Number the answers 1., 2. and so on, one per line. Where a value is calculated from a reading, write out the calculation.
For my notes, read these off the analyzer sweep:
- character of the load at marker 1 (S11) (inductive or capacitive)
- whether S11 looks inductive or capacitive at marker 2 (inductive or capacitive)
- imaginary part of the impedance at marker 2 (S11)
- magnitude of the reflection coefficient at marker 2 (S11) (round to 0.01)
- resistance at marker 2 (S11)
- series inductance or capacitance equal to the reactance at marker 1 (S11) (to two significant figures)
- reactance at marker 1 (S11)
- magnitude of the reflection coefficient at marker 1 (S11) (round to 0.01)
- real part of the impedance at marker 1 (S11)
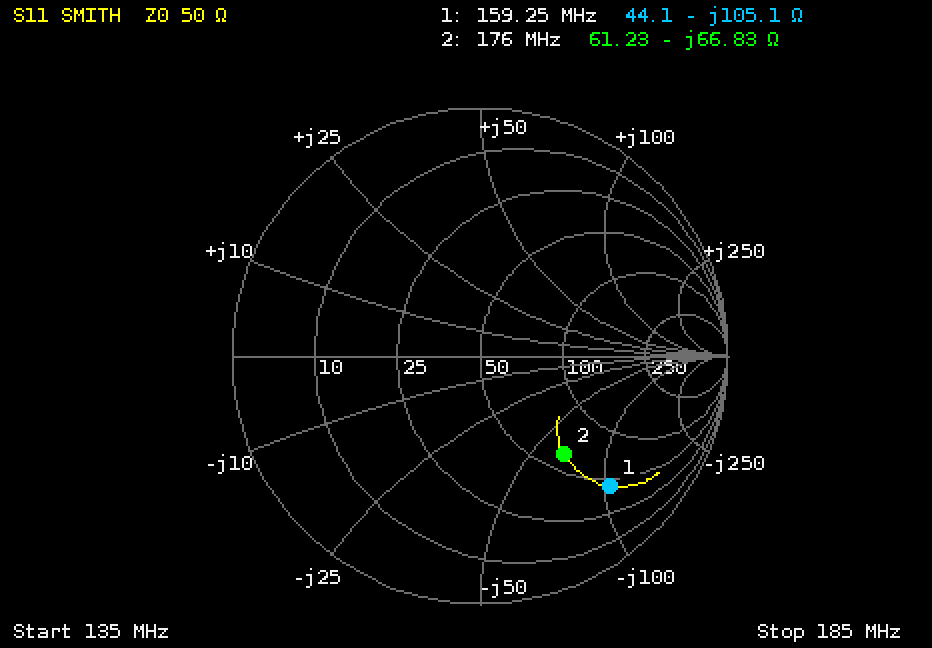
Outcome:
1. capacitive
2. capacitive
3. -66.83 Ω
4. 0.52
5. 61.23 Ω
6. C = 1/(2π × 159.25 MHz × 105.1 Ω) ≈ 9.5 pF
7. -105.1 Ω
8. 0.75
9. 44.1 Ω
